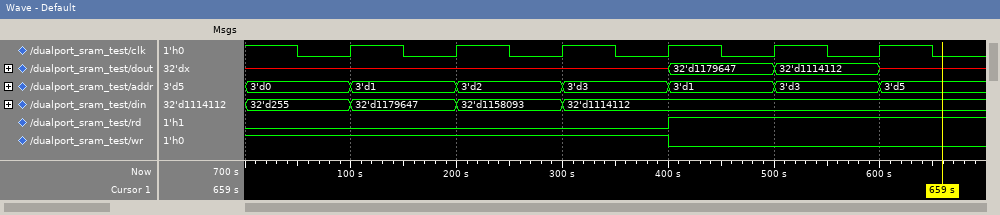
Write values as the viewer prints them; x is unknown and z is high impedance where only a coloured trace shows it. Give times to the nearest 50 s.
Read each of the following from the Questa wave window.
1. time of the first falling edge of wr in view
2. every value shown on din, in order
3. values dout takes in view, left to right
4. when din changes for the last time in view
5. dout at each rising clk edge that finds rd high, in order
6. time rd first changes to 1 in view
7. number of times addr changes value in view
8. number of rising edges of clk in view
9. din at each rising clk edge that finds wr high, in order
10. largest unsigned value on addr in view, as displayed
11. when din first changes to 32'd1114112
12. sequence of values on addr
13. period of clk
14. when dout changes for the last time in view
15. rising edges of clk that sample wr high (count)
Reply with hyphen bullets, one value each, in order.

- 400 s
- 32'd255, 32'd1179647, 32'd1158093, 32'd1114112
- x, 32'd1179647, 32'd1114112, x
- 300 s
- 32'd1179647, 32'd1114112
- 400 s
- 6
- 6
- 32'd255, 32'd1179647, 32'd1158093, 32'd1114112
- 3'd5
- 300 s
- 3'd0, 3'd1, 3'd2, 3'd3, 3'd1, 3'd3, 3'd5
- 100 s
- 600 s
- 4
